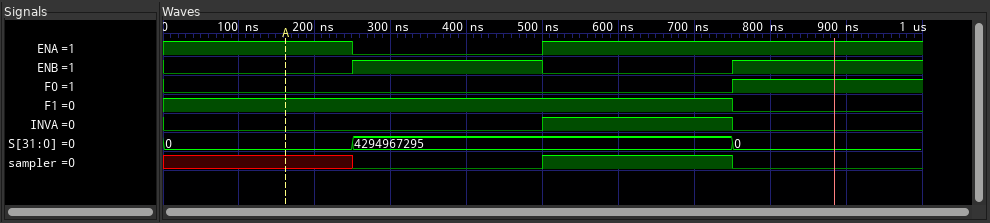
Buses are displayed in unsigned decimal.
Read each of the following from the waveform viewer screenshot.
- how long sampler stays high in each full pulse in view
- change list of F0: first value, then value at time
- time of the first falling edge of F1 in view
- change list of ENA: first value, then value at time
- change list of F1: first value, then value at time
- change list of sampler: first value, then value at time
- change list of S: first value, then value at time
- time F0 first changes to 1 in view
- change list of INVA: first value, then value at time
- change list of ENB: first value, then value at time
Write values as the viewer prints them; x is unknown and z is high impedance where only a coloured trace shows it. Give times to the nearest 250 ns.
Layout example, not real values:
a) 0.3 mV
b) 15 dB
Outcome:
a) 250 ns
b) 0, 1 at 750 ns
c) 750 ns
d) 1, 0 at 250 ns, 1 at 500 ns
e) 1, 0 at 750 ns
f) x, 0 at 250 ns, 1 at 500 ns, 0 at 750 ns
g) 0, 4294967295 at 250 ns, 0 at 750 ns
h) 750 ns
i) 0, 1 at 500 ns, 0 at 750 ns
j) 0, 1 at 250 ns, 0 at 500 ns, 1 at 750 ns
